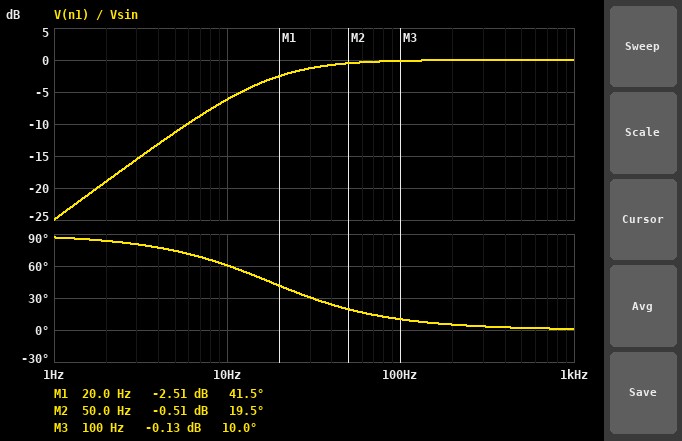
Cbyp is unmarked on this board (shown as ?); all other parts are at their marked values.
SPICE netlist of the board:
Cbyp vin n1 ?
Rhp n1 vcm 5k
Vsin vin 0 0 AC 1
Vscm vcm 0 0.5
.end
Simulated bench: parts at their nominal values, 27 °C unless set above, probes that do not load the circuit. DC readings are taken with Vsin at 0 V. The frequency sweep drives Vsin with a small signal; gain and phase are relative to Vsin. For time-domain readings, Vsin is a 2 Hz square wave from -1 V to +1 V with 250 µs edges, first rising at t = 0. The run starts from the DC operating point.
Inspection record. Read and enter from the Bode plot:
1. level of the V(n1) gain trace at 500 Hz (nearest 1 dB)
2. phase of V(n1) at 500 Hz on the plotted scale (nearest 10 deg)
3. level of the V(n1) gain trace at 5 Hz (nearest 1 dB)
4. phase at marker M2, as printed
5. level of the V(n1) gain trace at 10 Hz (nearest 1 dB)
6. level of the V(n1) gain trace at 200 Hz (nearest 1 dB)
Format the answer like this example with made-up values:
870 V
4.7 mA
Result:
0 dB
0 deg
-11 dB
19.5 deg
-6 dB
0 dB
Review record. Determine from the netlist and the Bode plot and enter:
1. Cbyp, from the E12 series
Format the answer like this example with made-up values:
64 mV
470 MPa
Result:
1.8 µF
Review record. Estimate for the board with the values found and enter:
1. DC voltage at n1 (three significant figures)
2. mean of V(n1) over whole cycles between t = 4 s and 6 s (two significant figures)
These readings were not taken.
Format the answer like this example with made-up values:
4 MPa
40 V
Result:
500 mV
500 mV
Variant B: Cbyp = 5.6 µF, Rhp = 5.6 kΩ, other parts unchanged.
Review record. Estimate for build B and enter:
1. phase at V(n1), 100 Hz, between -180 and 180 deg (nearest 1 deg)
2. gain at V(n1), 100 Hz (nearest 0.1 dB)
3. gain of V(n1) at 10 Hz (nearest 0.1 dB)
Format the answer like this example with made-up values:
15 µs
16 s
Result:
3 deg
0 dB
-1.0 dB
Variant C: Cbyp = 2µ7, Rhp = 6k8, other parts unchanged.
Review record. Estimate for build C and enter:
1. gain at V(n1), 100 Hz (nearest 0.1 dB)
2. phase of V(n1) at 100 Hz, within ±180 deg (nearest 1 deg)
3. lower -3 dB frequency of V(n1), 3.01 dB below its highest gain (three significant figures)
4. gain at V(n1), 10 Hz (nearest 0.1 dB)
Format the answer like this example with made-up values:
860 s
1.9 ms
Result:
0 dB
5 deg
8.67 Hz
-2.4 dB
